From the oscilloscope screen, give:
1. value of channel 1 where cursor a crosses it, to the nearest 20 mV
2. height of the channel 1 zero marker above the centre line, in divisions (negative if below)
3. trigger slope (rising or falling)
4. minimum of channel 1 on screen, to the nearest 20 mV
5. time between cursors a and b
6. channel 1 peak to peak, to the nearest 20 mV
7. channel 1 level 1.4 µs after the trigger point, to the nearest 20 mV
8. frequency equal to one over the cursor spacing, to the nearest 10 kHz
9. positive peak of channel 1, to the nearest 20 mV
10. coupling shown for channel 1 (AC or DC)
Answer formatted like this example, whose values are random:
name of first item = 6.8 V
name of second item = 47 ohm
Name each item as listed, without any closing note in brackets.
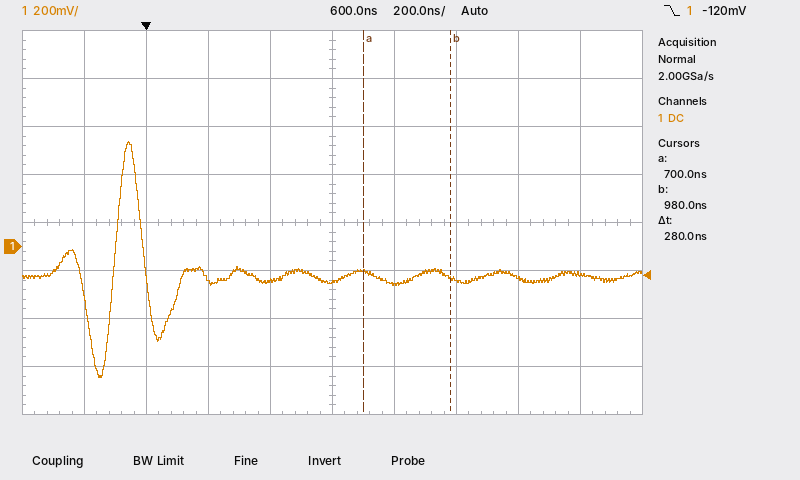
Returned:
value of channel 1 where cursor a crosses it, to the nearest 20 mV = -100 mV
height of the channel 1 zero marker above the centre line, in divisions = -0.5 div
trigger slope = falling
minimum of channel 1 on screen, to the nearest 20 mV = -540 mV
time between cursors a and b = 280 ns
channel 1 peak to peak, to the nearest 20 mV = 980 mV
channel 1 level 1.4 µs after the trigger point, to the nearest 20 mV = -120 mV
frequency equal to one over the cursor spacing, to the nearest 10 kHz = 3.57 MHz
positive peak of channel 1, to the nearest 20 mV = 440 mV
coupling shown for channel 1 = DC
